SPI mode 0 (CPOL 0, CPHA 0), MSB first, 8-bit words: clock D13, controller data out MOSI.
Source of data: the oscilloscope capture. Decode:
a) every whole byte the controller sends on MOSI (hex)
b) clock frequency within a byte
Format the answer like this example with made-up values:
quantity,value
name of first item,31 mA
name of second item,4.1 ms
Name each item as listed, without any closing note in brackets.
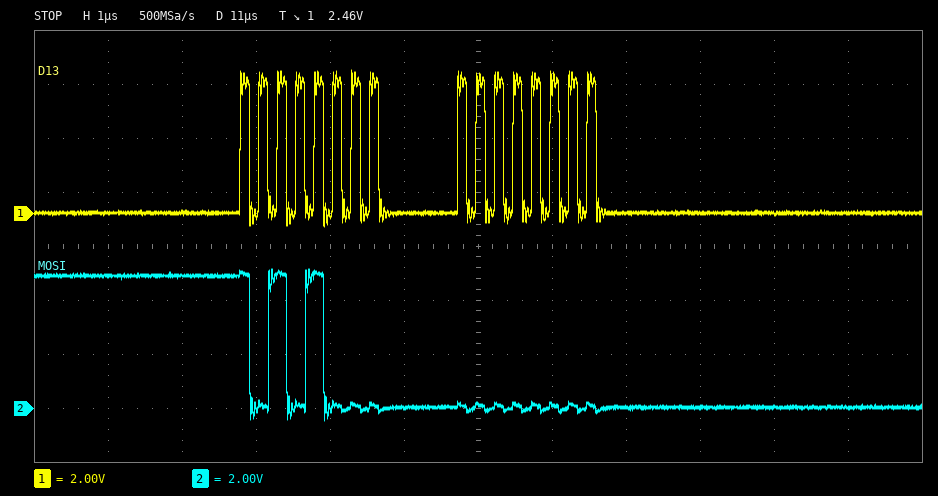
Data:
quantity,value
every whole byte the controller sends on MOSI,A8 00
clock frequency within a byte,4 MHz
